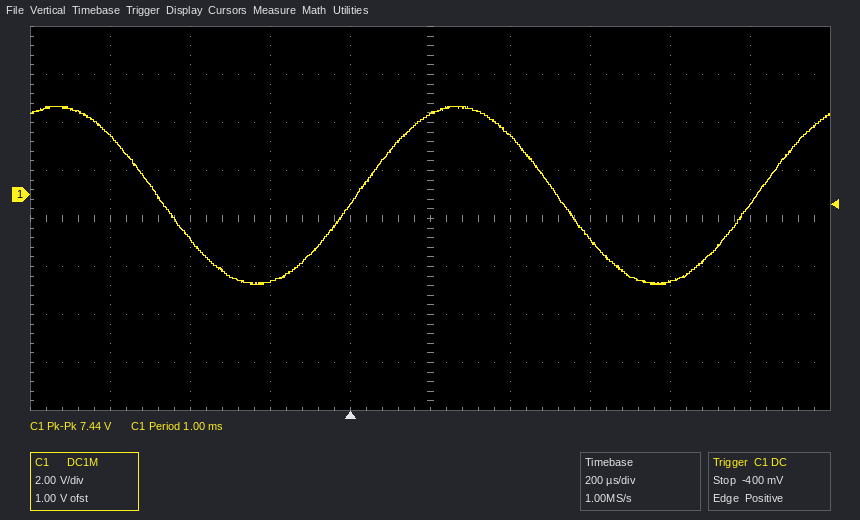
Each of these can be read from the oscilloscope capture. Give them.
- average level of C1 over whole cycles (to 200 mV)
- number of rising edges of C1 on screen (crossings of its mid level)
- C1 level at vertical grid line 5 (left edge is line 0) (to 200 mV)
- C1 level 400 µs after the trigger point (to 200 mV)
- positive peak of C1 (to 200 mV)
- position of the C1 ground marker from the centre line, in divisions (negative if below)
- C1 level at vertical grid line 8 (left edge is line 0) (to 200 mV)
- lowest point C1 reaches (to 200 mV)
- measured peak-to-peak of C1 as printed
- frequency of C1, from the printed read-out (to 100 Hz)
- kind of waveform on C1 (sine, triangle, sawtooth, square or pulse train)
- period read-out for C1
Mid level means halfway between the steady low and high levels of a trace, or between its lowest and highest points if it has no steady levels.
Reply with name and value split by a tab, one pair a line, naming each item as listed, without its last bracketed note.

average level of C1 over whole cycles	0.0 V
number of rising edges of C1 on screen	2
C1 level at vertical grid line 5 (left edge is line 0)	3.4 V
C1 level 400 µs after the trigger point	2.4 V
positive peak of C1	3.6 V
position of the C1 ground marker from the centre line, in divisions	+0.5 div
C1 level at vertical grid line 8 (left edge is line 0)	-3.6 V
lowest point C1 reaches	-3.8 V
measured peak-to-peak of C1 as printed	7.44 V
frequency of C1, from the printed read-out	1.0 kHz
kind of waveform on C1	sine
period read-out for C1	1.00 ms
